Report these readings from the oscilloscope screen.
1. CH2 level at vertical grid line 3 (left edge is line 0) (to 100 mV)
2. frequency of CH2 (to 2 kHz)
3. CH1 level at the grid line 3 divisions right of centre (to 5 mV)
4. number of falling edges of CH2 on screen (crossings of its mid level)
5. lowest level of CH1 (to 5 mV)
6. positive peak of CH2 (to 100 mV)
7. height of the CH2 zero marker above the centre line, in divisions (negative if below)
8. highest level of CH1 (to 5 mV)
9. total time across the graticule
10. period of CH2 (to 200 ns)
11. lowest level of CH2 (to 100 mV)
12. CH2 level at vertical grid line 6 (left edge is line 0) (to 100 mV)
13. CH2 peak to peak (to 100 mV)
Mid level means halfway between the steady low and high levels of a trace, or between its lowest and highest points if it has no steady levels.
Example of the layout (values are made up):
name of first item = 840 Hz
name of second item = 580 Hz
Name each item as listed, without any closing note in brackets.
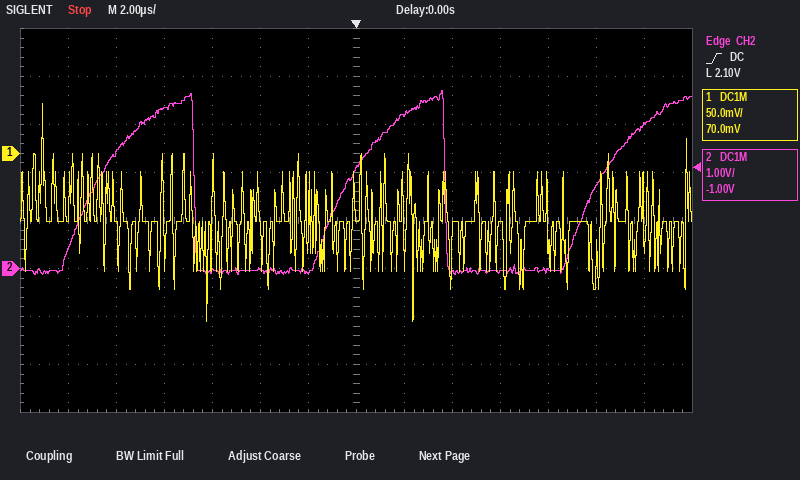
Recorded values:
CH2 level at vertical grid line 3 (left edge is line 0) = 3.3 V
frequency of CH2 = 96 kHz
CH1 level at the grid line 3 divisions right of centre = -75 mV
number of falling edges of CH2 on screen = 2
lowest level of CH1 = -175 mV
positive peak of CH2 = 3.7 V
height of the CH2 zero marker above the centre line, in divisions = -1.0 div
highest level of CH1 = 50 mV
total time across the graticule = 28 µs
period of CH2 = 10.4 µs
lowest level of CH2 = -100 mV
CH2 level at vertical grid line 6 (left edge is line 0) = -100 mV
CH2 peak to peak = 3.8 V
